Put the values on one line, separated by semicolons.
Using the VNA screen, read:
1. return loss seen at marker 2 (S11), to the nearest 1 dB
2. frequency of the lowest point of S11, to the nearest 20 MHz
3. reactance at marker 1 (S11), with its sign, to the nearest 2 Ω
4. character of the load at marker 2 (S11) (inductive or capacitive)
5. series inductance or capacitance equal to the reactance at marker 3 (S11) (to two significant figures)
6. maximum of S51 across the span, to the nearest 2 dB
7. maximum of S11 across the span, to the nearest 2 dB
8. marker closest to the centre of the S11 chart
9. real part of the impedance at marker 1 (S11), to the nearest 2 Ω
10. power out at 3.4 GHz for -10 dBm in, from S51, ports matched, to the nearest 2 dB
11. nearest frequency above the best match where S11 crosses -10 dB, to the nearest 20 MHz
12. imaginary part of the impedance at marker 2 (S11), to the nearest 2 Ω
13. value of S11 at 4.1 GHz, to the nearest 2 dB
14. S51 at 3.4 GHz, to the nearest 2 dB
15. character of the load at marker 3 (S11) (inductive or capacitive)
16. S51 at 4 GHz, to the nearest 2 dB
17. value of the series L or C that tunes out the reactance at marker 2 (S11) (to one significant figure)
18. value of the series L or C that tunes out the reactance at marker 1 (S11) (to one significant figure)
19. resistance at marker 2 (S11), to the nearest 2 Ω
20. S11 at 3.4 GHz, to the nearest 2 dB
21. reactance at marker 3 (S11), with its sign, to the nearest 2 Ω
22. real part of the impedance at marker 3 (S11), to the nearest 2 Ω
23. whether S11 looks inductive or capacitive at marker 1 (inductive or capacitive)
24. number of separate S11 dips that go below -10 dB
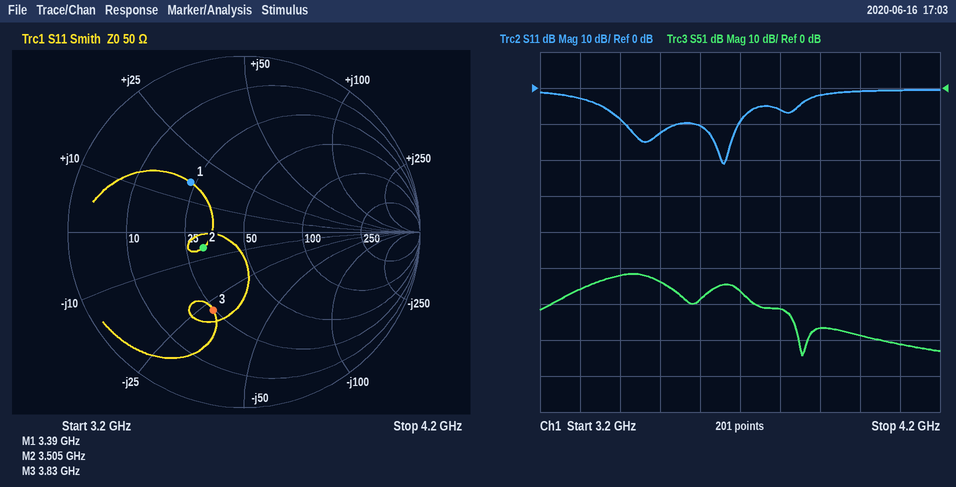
12 dB; 3.66 GHz; +16 Ω; capacitive; 1.5 pF; -52 dB; 0 dB; marker 2; 24 Ω; -62 dBm; 3.70 GHz; -6 Ω; 0 dB; -52 dB; capacitive; -68 dB; 300 pH; 3 pF; 30 Ω; -8 dB; -28 Ω; 24 Ω; inductive; 2
